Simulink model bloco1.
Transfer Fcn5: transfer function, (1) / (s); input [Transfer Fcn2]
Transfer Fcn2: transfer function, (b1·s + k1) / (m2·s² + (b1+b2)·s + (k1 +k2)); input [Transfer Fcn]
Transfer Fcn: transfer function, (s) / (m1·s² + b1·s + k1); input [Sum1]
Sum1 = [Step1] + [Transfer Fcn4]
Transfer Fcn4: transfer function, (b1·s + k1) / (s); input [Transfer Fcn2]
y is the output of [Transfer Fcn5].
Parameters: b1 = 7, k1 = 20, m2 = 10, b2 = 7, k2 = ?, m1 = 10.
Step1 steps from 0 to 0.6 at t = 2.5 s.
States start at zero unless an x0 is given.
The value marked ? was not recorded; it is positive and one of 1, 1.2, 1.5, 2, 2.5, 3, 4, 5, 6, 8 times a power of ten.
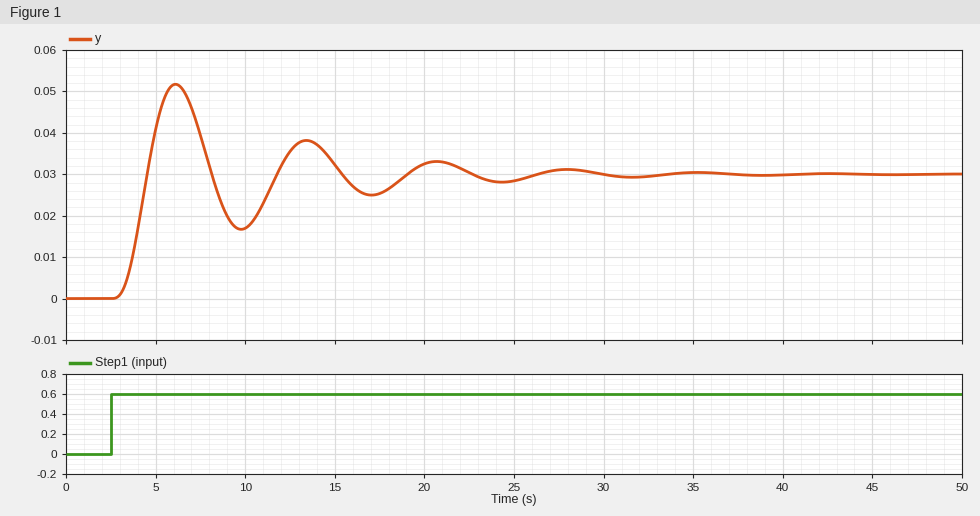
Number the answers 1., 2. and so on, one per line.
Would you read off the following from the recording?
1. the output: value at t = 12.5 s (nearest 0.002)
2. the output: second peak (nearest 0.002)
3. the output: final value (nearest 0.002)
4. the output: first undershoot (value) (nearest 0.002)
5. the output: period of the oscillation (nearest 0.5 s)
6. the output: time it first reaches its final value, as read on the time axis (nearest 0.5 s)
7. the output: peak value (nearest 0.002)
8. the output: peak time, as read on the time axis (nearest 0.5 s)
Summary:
1. 0.036
2. 0.038
3. 0.030
4. 0.016
5. 7.5 s
6. 4.5 s
7. 0.052
8. 6.0 s
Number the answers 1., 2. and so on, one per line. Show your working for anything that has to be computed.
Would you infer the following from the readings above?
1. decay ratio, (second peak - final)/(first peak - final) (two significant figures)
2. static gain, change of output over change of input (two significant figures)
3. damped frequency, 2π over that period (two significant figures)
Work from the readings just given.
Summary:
1. (0.038 - 0.03) / (0.052 - 0.03) = 0.36
2. (0.03 - 0) / (0.6 - 0) = 0.050
3. 2π / 7.5 = 0.84 rad/s
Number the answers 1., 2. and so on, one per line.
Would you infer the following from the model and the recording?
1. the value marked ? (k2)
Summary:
1. 20
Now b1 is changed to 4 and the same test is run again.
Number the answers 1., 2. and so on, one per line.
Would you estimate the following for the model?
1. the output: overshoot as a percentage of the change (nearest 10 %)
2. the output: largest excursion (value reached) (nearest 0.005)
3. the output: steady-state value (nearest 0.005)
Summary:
1. 80 %
2. 0.055
3. 0.030
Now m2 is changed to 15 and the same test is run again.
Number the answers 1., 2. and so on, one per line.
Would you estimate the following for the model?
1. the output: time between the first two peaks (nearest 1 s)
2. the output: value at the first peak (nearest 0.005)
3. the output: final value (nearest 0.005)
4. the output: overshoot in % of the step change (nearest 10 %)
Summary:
1. 8 s
2. 0.055
3. 0.030
4. 80 %
